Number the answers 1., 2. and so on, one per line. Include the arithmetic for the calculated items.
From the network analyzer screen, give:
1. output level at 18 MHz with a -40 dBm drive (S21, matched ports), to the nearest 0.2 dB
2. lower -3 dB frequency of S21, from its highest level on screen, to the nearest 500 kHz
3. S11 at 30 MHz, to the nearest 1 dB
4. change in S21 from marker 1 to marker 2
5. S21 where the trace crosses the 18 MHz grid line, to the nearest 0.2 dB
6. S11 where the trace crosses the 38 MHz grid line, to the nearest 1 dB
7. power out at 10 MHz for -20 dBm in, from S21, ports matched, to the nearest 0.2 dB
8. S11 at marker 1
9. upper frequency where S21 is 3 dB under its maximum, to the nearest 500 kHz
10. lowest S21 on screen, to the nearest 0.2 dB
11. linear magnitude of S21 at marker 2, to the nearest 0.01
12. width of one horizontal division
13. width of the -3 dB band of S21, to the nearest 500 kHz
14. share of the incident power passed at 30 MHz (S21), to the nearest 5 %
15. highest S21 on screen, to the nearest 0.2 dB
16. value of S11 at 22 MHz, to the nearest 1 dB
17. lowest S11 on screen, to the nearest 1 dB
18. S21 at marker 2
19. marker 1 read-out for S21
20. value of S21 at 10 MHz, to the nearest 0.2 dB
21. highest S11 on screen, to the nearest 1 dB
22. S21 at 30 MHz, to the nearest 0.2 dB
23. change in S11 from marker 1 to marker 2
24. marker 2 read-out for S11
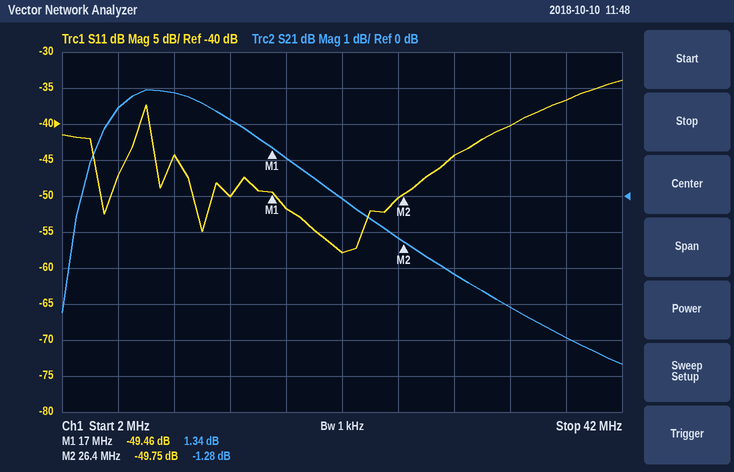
1. -40 dBm + (1.0 dB) = -39.0 dBm
2. 3.5 MHz
3. -44 dB
4. -1.28 − (1.34) = -2.62 dB
5. 1.0 dB
6. -37 dB
7. -20 dBm + (2.8 dB) = -17.2 dBm
8. -49.46 dB
9. 22.0 MHz
10. -4.6 dB
11. 10^(-1.28/20) ≈ 0.86
12. 4 MHz
13. 22.0 MHz − 3.5 MHz = 18.5 MHz
14. 10^(-2.2/10) ≈ 60 %
15. 3.0 dB
16. -58 dB
17. -58 dB
18. -1.28 dB
19. 1.34 dB
20. 2.8 dB
21. -34 dB
22. -2.2 dB
23. -49.75 − (-49.46) = -0.29 dB
24. -49.75 dB
